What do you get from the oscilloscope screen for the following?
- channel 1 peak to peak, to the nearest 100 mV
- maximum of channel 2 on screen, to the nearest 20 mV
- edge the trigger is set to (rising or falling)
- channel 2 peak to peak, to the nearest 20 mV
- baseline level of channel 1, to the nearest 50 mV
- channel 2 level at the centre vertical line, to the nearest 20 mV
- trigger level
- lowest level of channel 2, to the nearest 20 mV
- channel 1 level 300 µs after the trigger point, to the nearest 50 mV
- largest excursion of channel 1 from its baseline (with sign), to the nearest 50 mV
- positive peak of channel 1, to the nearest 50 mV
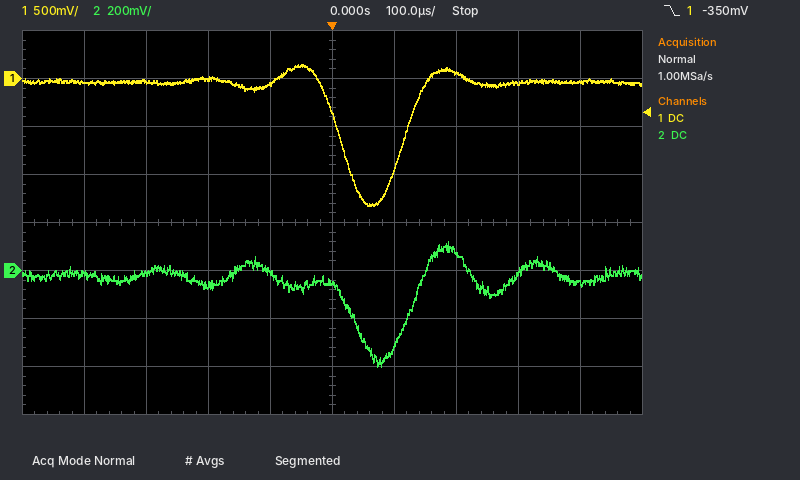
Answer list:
1.50 V
120 mV
falling
520 mV
-50 mV
-60 mV
-350 mV
-400 mV
-50 mV
-1.30 V
150 mV
